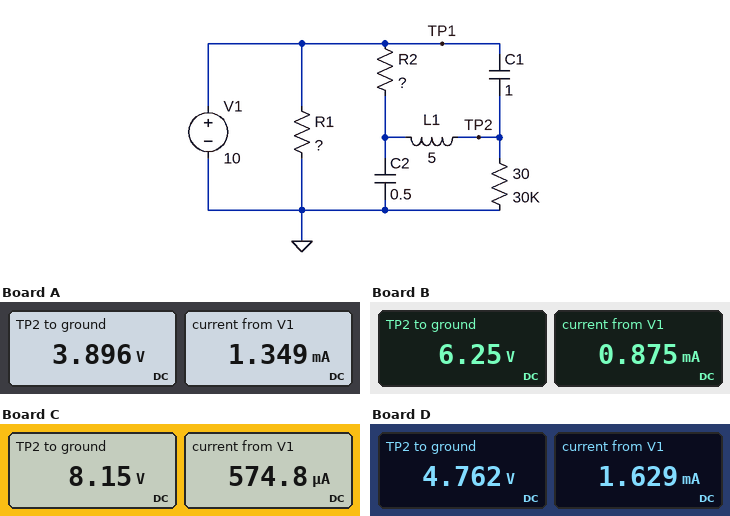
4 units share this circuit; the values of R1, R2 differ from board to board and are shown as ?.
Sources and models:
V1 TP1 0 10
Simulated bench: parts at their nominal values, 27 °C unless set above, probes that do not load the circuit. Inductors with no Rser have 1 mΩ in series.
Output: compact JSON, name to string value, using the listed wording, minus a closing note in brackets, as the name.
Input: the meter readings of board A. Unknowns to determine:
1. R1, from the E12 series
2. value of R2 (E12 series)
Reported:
{"R1, from the E12 series": "8.2 kΩ", "value of R2": "47 kΩ"}
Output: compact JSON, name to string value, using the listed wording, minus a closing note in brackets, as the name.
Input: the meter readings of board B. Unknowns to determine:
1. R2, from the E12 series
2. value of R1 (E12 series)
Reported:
{"R2, from the E12 series": "18 kΩ", "value of R1": "15 kΩ"}
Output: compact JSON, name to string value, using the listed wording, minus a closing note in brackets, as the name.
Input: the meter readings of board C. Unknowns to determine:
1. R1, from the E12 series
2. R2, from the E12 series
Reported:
{"R1, from the E12 series": "33 kΩ", "R2, from the E12 series": "6.8 kΩ"}
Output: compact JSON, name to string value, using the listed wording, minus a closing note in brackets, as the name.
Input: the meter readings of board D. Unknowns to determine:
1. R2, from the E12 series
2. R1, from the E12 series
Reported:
{"R2, from the E12 series": "33 kΩ", "R1, from the E12 series": "6.8 kΩ"}
